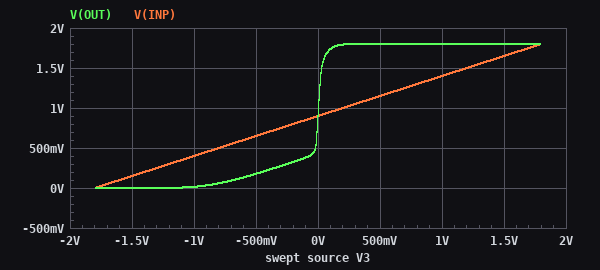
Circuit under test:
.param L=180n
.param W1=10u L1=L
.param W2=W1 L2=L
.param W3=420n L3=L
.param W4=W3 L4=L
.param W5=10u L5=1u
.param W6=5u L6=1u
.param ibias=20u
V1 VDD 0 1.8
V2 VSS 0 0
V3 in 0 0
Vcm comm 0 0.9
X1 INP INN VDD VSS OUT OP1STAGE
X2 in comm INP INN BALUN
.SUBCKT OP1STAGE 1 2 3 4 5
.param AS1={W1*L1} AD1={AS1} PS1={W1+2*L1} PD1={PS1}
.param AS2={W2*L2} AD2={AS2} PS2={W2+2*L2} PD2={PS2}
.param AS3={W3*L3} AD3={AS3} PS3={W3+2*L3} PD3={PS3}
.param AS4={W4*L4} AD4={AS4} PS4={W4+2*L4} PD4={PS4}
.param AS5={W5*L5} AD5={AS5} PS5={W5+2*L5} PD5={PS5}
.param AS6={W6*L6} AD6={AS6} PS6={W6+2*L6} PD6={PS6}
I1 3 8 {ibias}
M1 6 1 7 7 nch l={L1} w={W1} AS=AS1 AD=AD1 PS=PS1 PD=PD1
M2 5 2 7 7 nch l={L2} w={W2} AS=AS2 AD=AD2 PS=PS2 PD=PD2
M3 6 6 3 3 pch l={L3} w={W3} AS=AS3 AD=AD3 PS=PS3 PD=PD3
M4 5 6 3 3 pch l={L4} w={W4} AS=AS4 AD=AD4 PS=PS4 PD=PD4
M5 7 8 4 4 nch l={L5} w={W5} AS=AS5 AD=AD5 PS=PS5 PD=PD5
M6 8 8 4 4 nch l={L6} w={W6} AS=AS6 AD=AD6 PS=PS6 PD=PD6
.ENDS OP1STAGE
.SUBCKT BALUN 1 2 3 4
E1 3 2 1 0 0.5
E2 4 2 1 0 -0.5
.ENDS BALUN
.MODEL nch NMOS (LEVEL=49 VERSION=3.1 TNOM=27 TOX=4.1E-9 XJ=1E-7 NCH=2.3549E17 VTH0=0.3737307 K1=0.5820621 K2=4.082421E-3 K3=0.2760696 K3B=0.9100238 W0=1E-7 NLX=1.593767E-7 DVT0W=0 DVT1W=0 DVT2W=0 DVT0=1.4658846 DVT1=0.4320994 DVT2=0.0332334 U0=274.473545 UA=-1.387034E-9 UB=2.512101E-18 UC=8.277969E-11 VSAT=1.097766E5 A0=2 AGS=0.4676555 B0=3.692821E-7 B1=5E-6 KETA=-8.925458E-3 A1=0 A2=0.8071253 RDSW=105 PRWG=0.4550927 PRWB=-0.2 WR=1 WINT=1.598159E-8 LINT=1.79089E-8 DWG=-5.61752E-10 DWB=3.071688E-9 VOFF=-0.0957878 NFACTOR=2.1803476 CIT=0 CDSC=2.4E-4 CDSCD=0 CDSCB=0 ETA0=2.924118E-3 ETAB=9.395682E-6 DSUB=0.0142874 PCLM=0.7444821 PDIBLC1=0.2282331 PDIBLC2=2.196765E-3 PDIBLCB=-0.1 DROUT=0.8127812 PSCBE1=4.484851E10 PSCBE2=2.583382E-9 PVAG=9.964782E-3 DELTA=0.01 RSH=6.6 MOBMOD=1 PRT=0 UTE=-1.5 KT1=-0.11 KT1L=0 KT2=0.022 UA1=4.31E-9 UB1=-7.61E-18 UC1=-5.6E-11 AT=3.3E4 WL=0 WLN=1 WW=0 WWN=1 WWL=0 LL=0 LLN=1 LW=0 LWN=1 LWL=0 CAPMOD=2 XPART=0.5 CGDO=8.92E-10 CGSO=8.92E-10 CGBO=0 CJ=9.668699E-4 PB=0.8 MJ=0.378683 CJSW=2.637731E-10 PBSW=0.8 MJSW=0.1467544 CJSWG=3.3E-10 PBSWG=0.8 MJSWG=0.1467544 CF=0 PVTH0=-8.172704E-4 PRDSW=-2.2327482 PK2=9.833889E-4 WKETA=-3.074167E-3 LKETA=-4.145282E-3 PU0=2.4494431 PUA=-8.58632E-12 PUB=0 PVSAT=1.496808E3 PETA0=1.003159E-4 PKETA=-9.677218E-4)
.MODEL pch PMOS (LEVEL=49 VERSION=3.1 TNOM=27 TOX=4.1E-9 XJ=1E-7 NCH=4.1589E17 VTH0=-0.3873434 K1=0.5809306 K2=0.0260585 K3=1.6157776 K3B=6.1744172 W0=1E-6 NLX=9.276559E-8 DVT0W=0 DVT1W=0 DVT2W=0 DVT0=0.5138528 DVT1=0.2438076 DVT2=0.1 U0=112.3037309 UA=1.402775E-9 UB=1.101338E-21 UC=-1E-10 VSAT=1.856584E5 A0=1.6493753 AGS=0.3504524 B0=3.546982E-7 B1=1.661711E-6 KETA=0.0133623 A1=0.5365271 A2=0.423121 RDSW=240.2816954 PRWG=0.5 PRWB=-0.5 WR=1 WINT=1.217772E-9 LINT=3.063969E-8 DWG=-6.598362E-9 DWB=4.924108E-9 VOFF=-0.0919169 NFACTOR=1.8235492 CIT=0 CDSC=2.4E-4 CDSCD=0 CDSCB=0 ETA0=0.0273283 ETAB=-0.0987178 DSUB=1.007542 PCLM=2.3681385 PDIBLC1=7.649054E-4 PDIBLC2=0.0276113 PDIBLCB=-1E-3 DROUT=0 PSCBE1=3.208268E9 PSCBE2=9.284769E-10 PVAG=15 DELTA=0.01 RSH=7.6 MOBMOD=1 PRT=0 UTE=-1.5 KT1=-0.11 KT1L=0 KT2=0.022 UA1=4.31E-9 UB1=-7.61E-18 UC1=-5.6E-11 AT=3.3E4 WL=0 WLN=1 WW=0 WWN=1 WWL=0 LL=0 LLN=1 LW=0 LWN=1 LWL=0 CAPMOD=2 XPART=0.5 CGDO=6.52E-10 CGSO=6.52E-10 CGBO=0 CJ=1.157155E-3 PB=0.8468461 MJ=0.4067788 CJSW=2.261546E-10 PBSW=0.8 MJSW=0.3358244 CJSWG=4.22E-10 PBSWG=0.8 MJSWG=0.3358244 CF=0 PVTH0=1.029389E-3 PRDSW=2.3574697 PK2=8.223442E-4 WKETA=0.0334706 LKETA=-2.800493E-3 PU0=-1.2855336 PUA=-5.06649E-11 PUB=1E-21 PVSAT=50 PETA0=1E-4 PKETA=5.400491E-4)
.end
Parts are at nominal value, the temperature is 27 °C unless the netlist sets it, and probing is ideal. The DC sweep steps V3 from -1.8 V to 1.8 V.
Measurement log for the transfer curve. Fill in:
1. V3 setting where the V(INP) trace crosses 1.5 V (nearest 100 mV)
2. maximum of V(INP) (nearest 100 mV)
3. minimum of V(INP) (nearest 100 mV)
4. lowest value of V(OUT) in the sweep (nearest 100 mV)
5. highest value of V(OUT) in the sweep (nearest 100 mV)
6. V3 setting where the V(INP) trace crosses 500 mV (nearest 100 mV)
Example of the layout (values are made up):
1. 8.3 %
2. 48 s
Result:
1. 1.2 V
2. 1.8 V
3. 0 V
4. 0 V
5. 1.8 V
6. -800 mV
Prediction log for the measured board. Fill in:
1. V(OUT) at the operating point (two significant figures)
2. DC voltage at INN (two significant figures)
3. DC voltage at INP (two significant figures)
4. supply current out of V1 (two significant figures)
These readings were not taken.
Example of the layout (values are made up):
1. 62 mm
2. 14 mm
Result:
1. 900 mV
2. 900 mV
3. 900 mV
4. 59 µA
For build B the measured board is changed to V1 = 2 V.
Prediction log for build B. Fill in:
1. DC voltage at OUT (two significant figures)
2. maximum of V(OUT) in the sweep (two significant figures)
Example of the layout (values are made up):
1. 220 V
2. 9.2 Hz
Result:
1. 1.1 V
2. 2.0 V
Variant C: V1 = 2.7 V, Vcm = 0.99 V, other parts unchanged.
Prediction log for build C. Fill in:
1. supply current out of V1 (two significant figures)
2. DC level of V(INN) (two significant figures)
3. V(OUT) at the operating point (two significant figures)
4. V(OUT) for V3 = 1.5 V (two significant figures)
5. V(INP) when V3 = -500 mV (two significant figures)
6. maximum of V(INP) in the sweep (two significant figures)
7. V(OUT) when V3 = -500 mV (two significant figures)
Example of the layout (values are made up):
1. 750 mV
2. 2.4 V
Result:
1. 60 µA
2. 990 mV
3. 1.8 V
4. 2.7 V
5. 740 mV
6. 1.9 V
7. 290 mV
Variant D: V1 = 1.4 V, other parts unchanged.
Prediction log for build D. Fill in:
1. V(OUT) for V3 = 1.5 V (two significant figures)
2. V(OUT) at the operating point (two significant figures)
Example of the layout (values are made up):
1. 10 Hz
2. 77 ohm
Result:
1. 1.4 V
2. 500 mV
